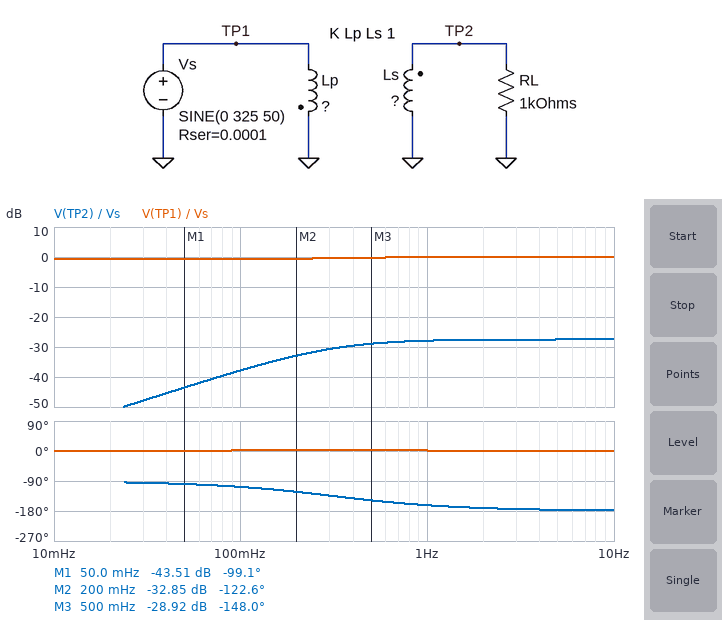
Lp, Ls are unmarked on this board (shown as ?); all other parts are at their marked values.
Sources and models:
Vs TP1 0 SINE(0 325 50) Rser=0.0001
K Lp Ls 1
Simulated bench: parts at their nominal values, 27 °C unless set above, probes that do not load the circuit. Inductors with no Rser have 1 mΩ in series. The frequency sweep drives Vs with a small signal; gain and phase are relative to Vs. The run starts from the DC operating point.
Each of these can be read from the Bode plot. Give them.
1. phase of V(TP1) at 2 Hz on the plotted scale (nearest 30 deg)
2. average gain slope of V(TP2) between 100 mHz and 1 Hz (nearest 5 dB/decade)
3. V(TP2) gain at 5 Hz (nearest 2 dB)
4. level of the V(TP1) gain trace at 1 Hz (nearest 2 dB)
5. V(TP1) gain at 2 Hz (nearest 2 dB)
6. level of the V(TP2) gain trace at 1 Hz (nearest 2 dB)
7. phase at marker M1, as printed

0 deg
10 dB/decade
-28 dB
0 dB
0 dB
-28 dB
-99.1 deg
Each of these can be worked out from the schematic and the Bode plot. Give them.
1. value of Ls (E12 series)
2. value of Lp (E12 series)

1 µH
560 µH
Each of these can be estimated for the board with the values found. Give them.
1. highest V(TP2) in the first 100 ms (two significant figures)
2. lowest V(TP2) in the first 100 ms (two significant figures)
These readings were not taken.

14 V
-14 V
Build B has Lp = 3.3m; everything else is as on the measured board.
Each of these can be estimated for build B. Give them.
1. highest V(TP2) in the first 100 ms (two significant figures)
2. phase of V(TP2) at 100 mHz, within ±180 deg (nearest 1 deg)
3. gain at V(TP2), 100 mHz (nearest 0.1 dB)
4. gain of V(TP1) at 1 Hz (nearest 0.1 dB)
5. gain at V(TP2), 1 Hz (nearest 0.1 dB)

5.7 V
-152 deg
-36.3 dB
0 dB
-35.2 dB
